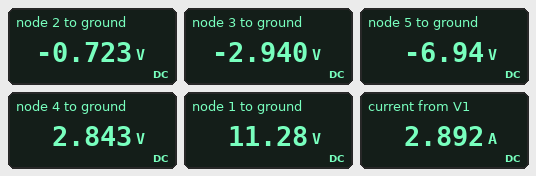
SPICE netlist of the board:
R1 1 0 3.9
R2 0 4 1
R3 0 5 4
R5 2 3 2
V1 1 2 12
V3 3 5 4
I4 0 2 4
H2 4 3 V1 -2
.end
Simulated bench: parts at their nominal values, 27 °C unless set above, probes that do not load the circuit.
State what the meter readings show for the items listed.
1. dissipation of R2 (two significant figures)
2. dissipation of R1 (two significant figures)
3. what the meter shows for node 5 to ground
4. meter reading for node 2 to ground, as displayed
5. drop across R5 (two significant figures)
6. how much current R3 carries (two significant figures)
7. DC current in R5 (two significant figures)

8.1 W
33 W
-6.94 V
-0.723 V
2.2 V
1.7 A
1.1 A
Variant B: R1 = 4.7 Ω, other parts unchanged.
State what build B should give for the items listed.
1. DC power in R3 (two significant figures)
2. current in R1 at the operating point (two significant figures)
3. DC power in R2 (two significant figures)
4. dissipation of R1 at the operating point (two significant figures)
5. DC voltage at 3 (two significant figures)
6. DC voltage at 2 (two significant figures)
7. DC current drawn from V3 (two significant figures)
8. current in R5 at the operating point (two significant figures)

10 W
2.6 A
8.7 W
33 W
-2.3 V
400 mV
1.6 A
1.4 A
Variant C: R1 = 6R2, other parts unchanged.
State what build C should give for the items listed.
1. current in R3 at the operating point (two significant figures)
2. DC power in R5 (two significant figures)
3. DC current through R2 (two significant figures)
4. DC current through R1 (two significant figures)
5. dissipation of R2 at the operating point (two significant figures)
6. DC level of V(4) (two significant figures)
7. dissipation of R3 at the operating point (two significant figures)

1.4 A
6.0 W
3.1 A
2.3 A
9.6 W
3.1 V
7.4 W
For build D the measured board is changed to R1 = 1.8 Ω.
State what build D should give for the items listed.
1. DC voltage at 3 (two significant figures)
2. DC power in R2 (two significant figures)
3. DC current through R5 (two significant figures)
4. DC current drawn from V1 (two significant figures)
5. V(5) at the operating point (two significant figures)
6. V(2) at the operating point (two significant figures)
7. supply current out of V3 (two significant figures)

-5.3 V
6.0 W
130 mA
3.9 A
-9.3 V
-5.0 V
2.3 A
